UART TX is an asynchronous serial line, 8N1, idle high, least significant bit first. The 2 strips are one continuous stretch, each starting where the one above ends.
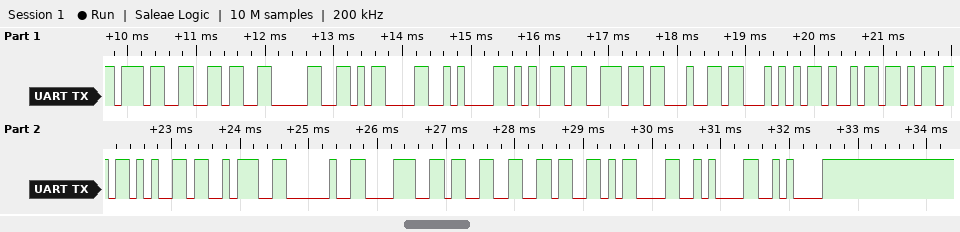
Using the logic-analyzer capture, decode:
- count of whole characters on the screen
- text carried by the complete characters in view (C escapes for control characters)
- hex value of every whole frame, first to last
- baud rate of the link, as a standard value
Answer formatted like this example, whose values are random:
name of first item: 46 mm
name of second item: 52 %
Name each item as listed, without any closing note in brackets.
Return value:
count of whole characters on the screen: 20
text carried by the complete characters in view: "760\r\nendTime: 836\r\n\n"
hex value of every whole frame, first to last: 0x37 0x36 0x30 0x0D 0x0A 0x65 0x6E 0x64 0x54 0x69 0x6D 0x65 0x3A 0x20 0x38 0x33 0x36 0x0D 0x0A 0x0A
baud rate of the link, as a standard value: 9600 baud
